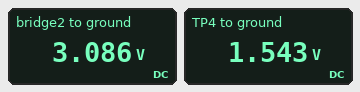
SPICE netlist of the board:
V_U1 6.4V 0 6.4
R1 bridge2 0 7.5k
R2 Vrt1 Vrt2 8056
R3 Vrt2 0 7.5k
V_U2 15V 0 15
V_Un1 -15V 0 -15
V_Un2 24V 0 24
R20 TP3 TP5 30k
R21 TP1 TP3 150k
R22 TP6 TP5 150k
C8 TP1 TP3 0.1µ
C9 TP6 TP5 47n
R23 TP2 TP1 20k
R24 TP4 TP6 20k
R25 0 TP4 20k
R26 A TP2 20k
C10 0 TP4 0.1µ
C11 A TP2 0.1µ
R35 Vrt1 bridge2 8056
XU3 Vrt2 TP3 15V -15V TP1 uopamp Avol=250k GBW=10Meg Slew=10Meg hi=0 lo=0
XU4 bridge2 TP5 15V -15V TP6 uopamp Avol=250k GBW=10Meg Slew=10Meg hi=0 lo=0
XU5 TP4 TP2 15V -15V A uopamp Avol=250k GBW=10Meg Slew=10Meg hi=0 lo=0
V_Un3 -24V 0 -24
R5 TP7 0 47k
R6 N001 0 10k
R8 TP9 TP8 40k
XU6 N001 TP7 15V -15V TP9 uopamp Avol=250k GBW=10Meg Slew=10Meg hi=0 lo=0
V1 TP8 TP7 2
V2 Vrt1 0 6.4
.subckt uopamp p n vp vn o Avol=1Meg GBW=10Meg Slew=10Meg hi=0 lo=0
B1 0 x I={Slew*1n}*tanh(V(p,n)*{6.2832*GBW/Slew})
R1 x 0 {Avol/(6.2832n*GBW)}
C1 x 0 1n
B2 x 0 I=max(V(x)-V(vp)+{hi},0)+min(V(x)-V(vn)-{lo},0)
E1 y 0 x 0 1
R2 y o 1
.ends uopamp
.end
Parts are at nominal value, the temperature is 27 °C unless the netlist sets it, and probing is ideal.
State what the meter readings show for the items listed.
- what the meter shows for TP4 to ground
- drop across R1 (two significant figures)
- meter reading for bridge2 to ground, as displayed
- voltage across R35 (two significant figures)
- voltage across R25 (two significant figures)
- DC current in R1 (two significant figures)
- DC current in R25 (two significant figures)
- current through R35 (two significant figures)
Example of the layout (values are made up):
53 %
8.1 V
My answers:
1.543 V
3.1 V
3.086 V
3.3 V
1.5 V
410 µA
77 µA
410 µA
